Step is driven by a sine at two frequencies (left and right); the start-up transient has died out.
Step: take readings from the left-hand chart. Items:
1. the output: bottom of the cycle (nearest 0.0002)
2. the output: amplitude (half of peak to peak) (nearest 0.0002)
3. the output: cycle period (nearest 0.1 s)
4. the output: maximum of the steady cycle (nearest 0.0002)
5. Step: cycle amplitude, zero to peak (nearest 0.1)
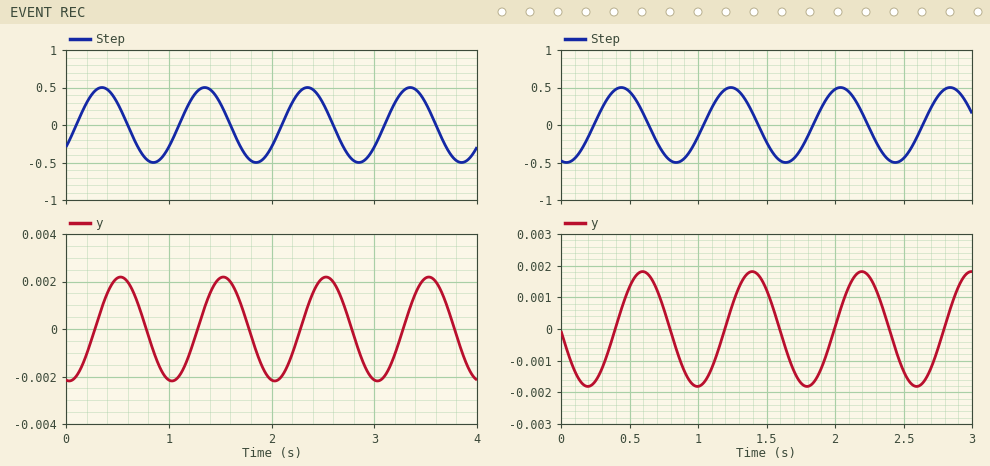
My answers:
-0.0022
0.0022
1.0 s
0.0022
0.5
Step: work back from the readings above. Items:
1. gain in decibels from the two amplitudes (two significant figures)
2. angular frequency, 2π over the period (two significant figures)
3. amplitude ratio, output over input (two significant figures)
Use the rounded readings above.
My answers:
-47 dB
6.3 rad/s
0.0044
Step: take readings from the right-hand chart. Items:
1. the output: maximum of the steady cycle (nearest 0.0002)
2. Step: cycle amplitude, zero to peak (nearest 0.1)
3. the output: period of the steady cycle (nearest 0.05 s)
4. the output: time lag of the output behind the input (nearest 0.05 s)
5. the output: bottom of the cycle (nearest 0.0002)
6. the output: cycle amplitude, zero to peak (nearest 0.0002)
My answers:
0.0018
0.5
0.80 s
0.15 s
-0.0018
0.0018
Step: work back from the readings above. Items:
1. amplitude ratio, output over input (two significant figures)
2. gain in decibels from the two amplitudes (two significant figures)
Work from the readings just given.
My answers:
0.0036
-49 dB
